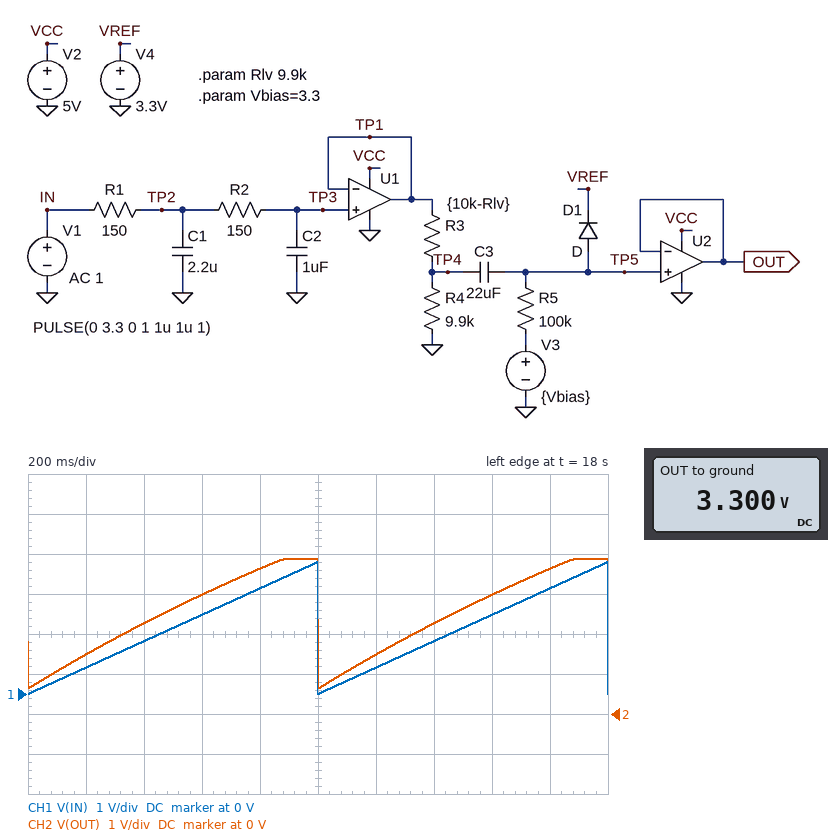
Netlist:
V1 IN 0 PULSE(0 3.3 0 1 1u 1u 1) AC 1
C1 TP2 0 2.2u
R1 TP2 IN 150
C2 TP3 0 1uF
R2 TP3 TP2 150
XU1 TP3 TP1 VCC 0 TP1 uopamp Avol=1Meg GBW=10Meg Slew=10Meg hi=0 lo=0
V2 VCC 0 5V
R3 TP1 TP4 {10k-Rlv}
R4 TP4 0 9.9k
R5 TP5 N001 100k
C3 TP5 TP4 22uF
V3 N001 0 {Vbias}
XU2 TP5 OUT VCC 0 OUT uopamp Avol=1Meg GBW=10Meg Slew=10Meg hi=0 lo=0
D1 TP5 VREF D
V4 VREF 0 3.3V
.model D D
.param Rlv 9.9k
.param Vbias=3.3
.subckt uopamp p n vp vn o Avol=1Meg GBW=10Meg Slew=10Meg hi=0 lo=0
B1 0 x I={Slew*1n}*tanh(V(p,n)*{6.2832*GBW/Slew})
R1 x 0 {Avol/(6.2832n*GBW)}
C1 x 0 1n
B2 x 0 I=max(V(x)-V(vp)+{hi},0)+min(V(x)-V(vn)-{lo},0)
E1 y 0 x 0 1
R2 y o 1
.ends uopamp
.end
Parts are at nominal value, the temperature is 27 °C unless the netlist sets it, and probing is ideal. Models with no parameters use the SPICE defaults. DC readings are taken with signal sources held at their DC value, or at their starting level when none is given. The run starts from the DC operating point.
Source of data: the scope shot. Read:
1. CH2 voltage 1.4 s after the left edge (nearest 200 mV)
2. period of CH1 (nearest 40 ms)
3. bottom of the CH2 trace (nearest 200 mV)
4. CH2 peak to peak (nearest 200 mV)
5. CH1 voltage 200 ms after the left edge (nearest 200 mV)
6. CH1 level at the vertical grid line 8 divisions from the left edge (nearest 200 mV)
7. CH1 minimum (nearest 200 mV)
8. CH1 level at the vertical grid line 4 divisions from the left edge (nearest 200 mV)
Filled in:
2.2 V
1.00 s
600 mV
3.2 V
600 mV
2.0 V
0 V
2.6 V
